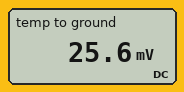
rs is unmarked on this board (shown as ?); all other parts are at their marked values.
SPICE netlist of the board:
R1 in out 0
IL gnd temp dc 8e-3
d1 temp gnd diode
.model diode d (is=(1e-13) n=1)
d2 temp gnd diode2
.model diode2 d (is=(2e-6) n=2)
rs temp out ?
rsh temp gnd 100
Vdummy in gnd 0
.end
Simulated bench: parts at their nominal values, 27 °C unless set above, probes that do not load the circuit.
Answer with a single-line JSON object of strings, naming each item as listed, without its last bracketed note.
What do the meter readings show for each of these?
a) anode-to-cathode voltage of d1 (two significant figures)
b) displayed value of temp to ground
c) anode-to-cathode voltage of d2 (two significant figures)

{"anode-to-cathode voltage of d1": "26 mV", "displayed value of temp to ground": "25.6 mV", "anode-to-cathode voltage of d2": "26 mV"}
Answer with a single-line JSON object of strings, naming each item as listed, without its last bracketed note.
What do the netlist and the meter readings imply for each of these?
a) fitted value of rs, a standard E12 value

{"fitted value of rs, a standard E12 value": "3.3 Ω"}
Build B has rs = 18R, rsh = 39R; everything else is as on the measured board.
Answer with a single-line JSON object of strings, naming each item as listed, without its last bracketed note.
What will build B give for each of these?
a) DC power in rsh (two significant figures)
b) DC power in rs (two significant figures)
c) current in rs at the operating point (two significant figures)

{"DC power in rsh": "250 µW", "DC power in rs": "540 µW", "current in rs at the operating point": "5.5 mA"}
